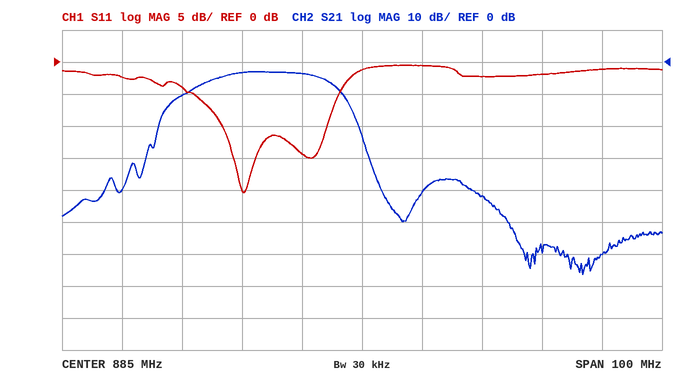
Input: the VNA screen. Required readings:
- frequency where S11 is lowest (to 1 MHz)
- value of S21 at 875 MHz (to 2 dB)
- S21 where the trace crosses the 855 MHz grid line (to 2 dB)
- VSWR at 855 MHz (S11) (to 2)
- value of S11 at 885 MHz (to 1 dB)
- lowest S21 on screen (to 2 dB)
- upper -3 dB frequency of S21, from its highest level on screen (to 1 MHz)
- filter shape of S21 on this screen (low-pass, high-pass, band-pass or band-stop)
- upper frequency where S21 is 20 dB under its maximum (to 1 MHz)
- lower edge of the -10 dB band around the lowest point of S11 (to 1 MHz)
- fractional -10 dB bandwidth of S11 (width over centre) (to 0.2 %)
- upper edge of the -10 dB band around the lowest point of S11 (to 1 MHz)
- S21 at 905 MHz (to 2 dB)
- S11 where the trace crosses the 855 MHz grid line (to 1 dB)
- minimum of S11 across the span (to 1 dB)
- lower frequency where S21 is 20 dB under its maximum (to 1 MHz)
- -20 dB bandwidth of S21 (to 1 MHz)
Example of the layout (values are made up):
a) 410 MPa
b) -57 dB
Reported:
a) 865 MHz
b) -4 dB
c) -10 dB
d) 4
e) -1 dB
f) -66 dB
g) 879 MHz
h) band-pass
i) 885 MHz
j) 862 MHz
k) 2.0 %
l) 879 MHz
m) -42 dB
n) -4 dB
o) -20 dB
p) 851 MHz
q) 34 MHz
